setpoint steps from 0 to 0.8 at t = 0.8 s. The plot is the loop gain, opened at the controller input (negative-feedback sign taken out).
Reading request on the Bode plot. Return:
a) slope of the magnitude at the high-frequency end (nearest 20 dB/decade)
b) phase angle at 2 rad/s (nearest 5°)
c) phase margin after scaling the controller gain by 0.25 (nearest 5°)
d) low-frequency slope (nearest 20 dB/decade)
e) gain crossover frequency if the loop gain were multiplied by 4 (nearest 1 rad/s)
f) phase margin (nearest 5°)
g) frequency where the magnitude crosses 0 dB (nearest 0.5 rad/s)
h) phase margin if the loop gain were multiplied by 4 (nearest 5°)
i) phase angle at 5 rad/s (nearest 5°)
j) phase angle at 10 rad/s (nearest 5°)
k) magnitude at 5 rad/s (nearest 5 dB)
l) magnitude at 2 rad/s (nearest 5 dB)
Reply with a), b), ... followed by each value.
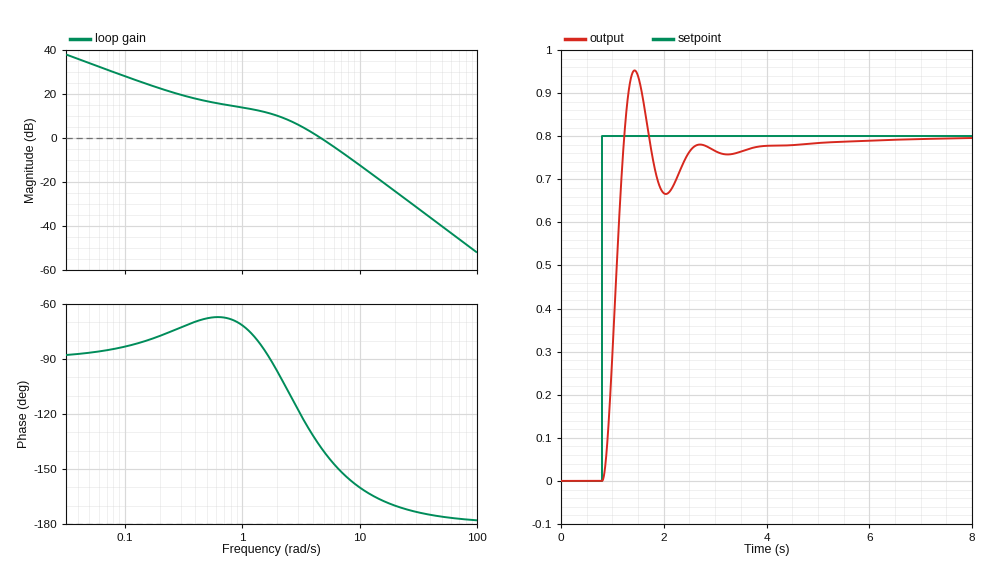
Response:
a) -40 dB/decade
b) -95°
c) 95°
d) -20 dB/decade
e) 10 rad/s
f) 40°
g) 4.5 rad/s
h) 20°
i) -140°
j) -160°
k) 0 dB
l) 10 dB
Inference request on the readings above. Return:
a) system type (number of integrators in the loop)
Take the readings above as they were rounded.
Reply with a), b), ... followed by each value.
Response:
a) 1
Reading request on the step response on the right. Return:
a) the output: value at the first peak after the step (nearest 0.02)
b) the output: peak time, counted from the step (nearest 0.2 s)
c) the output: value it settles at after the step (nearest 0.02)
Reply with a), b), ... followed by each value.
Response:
a) 0.96
b) 0.6 s
c) 0.80
